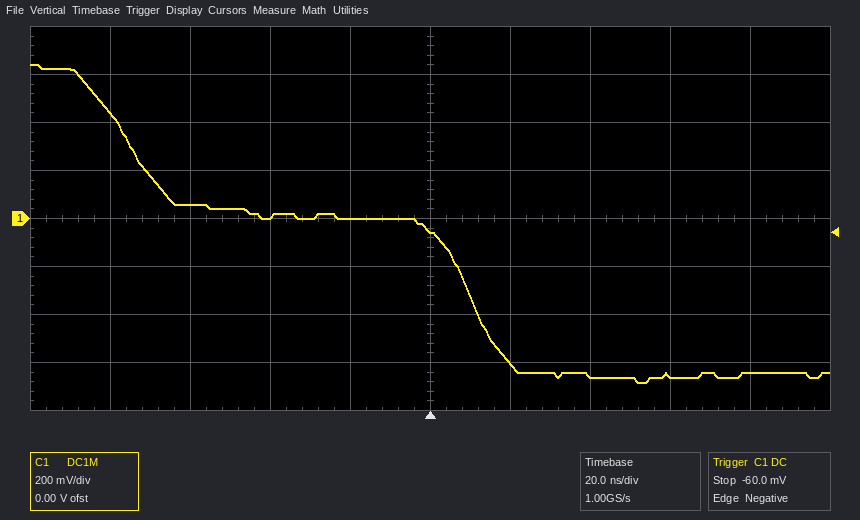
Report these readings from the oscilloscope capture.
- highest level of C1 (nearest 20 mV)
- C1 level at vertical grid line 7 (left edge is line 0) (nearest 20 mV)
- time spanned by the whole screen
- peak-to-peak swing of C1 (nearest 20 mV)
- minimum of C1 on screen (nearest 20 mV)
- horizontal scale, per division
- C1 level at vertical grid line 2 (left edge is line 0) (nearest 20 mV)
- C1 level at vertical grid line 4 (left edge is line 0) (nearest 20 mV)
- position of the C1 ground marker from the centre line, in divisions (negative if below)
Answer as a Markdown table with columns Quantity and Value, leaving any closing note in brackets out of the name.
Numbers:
| Quantity | Value |
|---|---|
| highest level of C1 | 640 mV |
| C1 level at vertical grid line 7 (left edge is line 0) | -660 mV |
| time spanned by the whole screen | 200 ns |
| peak-to-peak swing of C1 | 1.32 V |
| minimum of C1 on screen | -680 mV |
| horizontal scale, per division | 20 ns |
| C1 level at vertical grid line 2 (left edge is line 0) | 60 mV |
| C1 level at vertical grid line 4 (left edge is line 0) | 0 mV |
| position of the C1 ground marker from the centre line, in divisions | 0.0 div |
